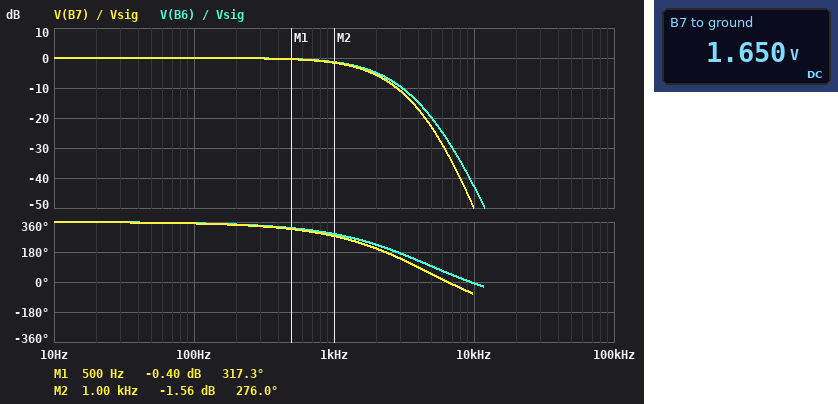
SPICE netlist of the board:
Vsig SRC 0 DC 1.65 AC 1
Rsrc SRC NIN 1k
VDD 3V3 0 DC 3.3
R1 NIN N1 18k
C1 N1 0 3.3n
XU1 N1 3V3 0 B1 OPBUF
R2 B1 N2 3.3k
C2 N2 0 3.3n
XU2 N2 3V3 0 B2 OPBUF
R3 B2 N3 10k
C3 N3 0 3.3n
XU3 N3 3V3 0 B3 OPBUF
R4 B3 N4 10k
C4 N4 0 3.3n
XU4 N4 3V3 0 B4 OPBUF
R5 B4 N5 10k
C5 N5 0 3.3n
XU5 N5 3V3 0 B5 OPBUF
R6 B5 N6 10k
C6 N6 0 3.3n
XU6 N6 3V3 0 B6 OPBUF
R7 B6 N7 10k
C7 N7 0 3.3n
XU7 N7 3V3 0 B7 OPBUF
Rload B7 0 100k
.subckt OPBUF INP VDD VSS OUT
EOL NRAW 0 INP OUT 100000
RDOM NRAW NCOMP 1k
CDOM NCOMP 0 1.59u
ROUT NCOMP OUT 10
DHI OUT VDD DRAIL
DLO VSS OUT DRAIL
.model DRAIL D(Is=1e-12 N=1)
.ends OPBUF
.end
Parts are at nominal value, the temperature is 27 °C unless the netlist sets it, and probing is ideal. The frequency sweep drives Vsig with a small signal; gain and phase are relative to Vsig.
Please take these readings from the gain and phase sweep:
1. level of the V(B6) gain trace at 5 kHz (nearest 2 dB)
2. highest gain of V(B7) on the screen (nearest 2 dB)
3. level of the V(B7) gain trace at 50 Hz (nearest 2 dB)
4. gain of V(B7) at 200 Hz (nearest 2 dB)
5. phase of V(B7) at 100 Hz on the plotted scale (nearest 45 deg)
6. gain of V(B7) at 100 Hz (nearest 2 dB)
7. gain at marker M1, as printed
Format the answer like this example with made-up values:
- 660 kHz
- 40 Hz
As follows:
- -20 dB
- 0 dB
- 0 dB
- 0 dB
- 360 deg
- 0 dB
- -0.40 dB
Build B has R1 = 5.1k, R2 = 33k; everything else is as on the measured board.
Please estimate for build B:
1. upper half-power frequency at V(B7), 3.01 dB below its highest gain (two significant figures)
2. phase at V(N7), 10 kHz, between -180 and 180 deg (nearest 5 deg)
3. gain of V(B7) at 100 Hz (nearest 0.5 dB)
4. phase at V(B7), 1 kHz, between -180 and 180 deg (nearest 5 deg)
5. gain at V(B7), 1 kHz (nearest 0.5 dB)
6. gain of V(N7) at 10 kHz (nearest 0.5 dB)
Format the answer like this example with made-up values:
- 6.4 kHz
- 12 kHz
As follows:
- 1.1 kHz
- -95 deg
- 0 dB
- -100 deg
- -2.5 dB
- -57.0 dB
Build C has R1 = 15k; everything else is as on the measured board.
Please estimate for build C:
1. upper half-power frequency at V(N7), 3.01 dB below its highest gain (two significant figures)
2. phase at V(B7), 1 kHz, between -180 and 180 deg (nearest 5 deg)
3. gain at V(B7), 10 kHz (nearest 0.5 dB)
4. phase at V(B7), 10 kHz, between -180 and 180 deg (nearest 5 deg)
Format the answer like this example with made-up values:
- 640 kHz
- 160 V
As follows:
- 1.5 kHz
- -80 deg
- -48.5 dB
- -70 deg
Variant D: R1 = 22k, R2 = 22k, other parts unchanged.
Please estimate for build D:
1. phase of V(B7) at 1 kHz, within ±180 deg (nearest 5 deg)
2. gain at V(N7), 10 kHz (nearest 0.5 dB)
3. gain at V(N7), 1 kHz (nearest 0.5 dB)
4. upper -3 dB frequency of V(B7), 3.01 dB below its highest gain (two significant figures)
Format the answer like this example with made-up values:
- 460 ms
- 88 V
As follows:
- -110 deg
- -63.5 dB
- -2.5 dB
- 1.1 kHz
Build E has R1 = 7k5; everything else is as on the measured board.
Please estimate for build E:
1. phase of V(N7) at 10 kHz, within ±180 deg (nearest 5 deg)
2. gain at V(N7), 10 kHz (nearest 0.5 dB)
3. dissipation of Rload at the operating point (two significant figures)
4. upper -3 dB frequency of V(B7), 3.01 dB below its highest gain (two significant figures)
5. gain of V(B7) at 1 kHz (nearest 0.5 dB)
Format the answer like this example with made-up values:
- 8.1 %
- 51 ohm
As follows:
- -55 deg
- -44.0 dB
- 27 µW
- 1.7 kHz
- -1.0 dB
